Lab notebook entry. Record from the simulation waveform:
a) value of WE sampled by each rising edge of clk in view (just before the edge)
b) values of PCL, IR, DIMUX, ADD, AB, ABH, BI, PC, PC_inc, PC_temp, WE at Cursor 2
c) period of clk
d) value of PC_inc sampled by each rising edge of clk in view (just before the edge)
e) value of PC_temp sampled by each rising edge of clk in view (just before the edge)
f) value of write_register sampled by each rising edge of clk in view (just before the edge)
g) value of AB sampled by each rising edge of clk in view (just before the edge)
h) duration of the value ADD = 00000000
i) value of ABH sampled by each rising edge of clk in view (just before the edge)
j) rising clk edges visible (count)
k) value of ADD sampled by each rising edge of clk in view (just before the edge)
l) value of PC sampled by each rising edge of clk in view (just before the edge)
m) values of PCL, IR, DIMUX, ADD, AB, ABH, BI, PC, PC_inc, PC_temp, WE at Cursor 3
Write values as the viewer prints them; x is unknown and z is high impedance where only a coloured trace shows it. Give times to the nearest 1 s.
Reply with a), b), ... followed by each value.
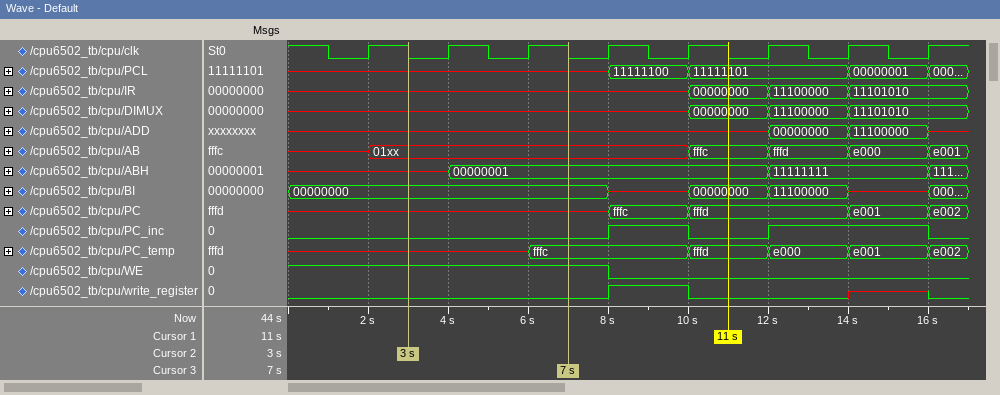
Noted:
a) 1 1 1 1 0 0 0 0
b) PCL=x, IR=x, DIMUX=x, ADD=x, AB=01xx, ABH=x, BI=00000000, PC=x, PC_inc=0, PC_temp=x, WE=1
c) 2 s
d) 0 0 0 0 1 0 1 1
e) x, x, x, fffc, fffc, fffd, e000, e001
f) 0 0 0 0 1 0 0 x
g) x, 01xx, 01xx, 01xx, 01xx, fffc, fffd, e000
h) 2 s
i) x, x, 00000001, 00000001, 00000001, 00000001, 11111111, 11111111
j) 8
k) x, x, x, x, x, x, 00000000, 11100000
l) x, x, x, x, fffc, fffd, fffd, e001
m) PCL=x, IR=x, DIMUX=x, ADD=x, AB=01xx, ABH=00000001, BI=00000000, PC=x, PC_inc=0, PC_temp=fffc, WE=1
